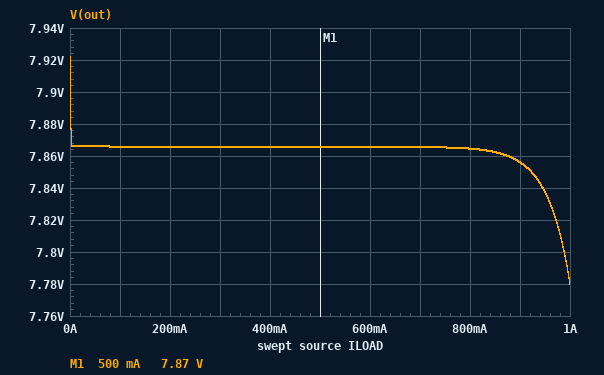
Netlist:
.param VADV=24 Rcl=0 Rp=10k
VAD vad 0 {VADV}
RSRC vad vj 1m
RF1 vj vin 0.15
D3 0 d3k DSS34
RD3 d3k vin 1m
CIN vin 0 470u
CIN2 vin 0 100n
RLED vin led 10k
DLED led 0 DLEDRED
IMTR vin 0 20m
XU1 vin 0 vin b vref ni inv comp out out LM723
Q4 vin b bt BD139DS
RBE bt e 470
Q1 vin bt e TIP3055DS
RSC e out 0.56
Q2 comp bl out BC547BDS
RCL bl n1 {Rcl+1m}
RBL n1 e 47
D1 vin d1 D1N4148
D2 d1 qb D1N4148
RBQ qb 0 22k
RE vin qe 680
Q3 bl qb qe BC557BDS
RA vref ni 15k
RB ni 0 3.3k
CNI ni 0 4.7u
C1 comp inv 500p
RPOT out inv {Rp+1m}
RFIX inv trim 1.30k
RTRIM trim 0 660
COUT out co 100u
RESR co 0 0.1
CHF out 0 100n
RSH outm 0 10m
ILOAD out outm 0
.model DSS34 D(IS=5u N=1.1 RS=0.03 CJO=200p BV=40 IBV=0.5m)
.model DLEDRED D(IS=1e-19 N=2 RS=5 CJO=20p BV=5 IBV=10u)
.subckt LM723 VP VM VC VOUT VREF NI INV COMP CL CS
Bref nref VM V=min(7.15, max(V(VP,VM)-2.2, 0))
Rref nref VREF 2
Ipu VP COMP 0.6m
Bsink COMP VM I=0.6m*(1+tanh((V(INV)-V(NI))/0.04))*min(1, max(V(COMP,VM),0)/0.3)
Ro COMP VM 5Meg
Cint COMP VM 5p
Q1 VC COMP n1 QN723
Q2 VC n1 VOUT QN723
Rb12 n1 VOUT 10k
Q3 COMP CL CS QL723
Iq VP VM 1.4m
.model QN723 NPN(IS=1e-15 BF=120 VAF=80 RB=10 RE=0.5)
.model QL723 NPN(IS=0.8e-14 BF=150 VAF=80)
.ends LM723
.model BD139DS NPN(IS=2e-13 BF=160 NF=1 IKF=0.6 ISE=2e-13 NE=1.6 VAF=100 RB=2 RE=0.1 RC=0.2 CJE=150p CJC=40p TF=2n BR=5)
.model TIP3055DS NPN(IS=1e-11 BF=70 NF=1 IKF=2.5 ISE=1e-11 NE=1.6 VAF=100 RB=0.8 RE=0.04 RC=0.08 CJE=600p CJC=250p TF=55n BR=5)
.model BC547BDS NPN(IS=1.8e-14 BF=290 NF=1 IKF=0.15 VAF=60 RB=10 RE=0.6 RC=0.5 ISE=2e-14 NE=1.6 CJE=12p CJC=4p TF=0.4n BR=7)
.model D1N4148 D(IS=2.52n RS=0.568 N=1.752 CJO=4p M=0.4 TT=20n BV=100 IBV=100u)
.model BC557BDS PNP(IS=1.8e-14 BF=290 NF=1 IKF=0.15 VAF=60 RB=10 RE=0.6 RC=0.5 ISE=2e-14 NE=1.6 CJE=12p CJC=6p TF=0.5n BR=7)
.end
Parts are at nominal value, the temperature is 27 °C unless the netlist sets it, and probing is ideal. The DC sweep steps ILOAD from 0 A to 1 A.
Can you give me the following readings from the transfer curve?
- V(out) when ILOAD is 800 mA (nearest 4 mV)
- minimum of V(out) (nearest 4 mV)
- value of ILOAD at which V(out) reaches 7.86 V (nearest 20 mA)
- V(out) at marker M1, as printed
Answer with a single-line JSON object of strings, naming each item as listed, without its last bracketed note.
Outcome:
{"V(out) when ILOAD is 800 mA": "7.864 V", "minimum of V(out)": "7.780 V", "value of ILOAD at which V(out) reaches 7.86 V": "880 mA", "V(out) at marker M1, as printed": "7.87 V"}
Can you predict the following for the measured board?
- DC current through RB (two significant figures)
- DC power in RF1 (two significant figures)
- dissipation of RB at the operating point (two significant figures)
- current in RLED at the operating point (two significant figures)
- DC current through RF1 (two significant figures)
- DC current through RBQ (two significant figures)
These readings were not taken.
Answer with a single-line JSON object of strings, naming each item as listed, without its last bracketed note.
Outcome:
{"DC current through RB": "390 µA", "DC power in RF1": "100 µW", "dissipation of RB at the operating point": "500 µW", "current in RLED at the operating point": "2.2 mA", "DC current through RF1": "26 mA", "DC current through RBQ": "1.0 mA"}
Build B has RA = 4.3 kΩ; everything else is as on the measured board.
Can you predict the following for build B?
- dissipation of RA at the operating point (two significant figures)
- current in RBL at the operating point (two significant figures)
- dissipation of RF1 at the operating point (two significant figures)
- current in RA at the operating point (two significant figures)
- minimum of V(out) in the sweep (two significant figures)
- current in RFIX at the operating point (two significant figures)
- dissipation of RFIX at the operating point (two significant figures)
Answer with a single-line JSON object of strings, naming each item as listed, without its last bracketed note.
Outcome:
{"dissipation of RA at the operating point": "3.8 mW", "current in RBL at the operating point": "790 µA", "dissipation of RF1 at the operating point": "110 µW", "current in RA at the operating point": "940 µA", "minimum of V(out) in the sweep": "19 V", "current in RFIX at the operating point": "1.6 mA", "dissipation of RFIX at the operating point": "3.3 mW"}
